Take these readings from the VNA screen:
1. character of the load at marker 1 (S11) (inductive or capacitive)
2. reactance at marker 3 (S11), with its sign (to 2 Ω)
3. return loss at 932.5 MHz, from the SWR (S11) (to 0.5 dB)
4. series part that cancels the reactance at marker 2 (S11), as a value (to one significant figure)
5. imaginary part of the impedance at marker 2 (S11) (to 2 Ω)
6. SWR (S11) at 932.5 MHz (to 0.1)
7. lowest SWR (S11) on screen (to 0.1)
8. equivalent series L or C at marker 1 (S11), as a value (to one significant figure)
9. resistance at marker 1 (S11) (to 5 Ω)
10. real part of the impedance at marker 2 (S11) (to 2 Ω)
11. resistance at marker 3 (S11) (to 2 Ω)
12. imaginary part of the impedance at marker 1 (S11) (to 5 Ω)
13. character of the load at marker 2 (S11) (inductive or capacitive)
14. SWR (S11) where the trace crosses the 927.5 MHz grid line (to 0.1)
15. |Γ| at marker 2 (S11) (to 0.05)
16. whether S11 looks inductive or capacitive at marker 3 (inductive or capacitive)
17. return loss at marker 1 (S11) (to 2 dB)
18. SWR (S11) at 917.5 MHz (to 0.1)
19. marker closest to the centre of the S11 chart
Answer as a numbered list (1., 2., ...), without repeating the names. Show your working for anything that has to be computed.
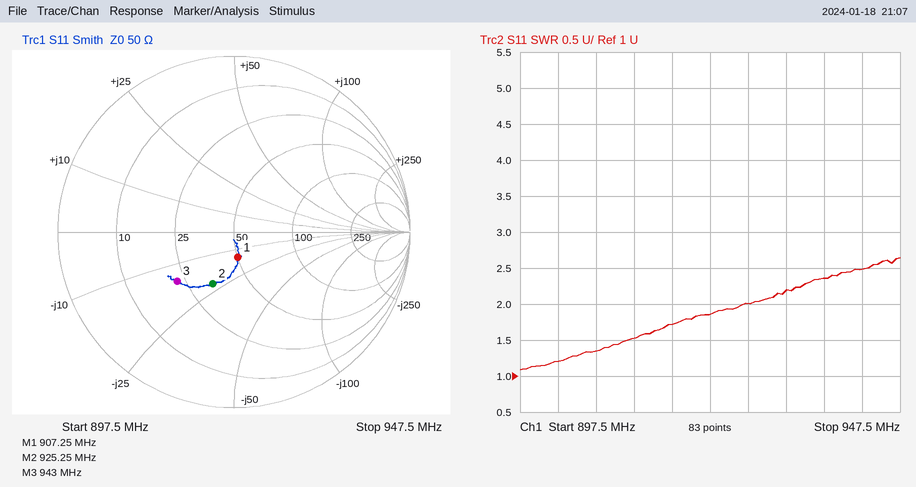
1. capacitive
2. -16 Ω
3. −20 log10((2.2 − 1)/(2.2 + 1)) ≈ 8.5 dB
4. L = 22 Ω/(2π × 925.25 MHz) ≈ 4 nH
5. -22 Ω
6. 2.2
7. 1.1
8. C = 1/(2π × 907.25 MHz × 15 Ω) ≈ 11.7 pF, so 10 pF to one significant figure
9. 50 Ω
10. 34 Ω
11. 22 Ω
12. -15 Ω
13. capacitive
14. 2.0
15. 0.30
16. capacitive
17. 16 dB
18. 1.7
19. marker 1
